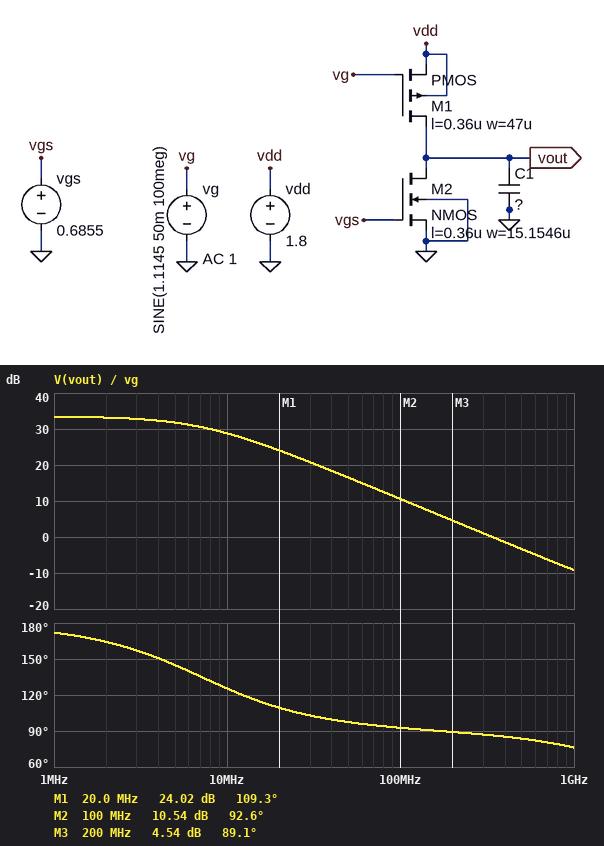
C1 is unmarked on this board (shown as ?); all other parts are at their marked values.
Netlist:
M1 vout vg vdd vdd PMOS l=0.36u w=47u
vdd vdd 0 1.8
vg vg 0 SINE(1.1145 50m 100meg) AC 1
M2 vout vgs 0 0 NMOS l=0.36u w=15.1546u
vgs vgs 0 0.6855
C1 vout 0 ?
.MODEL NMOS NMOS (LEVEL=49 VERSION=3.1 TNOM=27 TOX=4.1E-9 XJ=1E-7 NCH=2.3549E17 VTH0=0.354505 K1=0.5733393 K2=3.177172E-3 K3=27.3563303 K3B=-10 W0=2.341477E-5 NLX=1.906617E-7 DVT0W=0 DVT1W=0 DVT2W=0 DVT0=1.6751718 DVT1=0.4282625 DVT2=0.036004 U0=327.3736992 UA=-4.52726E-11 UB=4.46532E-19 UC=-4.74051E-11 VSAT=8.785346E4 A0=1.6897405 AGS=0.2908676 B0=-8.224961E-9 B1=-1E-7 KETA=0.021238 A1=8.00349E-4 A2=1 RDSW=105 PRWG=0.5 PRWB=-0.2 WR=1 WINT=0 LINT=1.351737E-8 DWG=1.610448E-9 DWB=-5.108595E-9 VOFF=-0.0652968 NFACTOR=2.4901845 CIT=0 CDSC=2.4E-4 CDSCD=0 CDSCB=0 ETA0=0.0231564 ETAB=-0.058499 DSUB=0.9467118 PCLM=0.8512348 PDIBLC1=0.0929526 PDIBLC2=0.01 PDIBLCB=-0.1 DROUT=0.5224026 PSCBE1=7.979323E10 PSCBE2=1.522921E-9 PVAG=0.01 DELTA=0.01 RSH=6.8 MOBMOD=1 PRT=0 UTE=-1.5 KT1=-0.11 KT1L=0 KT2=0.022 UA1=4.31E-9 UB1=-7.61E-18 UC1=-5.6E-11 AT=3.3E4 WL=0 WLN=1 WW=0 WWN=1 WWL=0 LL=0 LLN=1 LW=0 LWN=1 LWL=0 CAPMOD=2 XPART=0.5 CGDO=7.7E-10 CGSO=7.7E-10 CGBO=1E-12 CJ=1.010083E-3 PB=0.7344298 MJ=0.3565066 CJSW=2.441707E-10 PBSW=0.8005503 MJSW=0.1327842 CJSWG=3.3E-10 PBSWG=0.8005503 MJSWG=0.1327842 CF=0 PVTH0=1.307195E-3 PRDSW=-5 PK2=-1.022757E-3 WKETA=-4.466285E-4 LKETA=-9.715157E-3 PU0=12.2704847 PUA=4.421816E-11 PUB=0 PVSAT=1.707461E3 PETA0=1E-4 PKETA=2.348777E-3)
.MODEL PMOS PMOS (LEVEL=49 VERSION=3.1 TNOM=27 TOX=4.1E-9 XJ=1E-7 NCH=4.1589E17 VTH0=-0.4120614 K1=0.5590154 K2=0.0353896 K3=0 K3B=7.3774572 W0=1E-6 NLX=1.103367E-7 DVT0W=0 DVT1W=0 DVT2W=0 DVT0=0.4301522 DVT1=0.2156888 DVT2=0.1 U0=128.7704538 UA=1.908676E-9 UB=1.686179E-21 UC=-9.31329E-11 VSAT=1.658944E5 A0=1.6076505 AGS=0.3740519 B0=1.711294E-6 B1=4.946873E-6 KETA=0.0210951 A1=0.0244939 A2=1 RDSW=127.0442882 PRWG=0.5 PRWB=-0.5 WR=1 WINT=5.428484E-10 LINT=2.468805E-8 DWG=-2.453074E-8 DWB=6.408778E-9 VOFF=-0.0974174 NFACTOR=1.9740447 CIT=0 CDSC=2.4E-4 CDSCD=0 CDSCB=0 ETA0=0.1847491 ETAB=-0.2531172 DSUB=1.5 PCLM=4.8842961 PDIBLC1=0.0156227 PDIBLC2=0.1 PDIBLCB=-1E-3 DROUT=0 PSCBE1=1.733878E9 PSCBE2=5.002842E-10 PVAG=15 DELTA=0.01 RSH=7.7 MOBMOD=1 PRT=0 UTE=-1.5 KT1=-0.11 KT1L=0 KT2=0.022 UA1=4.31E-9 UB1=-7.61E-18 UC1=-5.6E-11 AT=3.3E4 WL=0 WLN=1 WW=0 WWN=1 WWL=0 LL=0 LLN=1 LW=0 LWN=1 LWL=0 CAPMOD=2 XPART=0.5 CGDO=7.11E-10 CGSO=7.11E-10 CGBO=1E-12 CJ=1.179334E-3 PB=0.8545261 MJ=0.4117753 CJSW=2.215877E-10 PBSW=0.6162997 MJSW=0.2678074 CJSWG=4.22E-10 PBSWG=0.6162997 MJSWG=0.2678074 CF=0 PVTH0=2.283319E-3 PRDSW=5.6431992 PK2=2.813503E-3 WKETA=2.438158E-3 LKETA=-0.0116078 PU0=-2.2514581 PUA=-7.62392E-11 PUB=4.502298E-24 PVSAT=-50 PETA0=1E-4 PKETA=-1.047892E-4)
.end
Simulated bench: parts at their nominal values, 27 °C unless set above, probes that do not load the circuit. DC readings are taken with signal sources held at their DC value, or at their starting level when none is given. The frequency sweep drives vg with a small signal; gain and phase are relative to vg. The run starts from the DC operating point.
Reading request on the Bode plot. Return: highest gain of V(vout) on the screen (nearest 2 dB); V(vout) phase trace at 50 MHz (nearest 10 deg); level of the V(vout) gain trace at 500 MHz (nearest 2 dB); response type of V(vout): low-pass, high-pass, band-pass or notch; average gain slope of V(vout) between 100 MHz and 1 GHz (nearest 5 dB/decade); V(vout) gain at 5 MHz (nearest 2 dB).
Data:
34 dB
100 deg
-4 dB
low-pass
-20 dB/decade
32 dB
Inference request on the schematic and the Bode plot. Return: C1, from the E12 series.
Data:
820 fF
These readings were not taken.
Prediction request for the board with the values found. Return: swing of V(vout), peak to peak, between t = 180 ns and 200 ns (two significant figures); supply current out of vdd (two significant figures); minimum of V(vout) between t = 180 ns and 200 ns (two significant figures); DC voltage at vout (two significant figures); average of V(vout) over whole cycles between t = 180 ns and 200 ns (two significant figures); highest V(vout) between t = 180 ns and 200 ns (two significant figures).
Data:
330 mV
220 µA
830 mV
880 mV
1.0 V
1.2 V
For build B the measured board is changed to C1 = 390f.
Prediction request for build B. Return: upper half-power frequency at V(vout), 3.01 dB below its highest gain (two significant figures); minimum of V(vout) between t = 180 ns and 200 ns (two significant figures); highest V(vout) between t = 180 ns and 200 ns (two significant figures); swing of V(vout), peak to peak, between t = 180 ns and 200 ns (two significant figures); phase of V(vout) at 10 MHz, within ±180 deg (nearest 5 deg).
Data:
14 MHz
680 mV
1.3 V
640 mV
145 deg
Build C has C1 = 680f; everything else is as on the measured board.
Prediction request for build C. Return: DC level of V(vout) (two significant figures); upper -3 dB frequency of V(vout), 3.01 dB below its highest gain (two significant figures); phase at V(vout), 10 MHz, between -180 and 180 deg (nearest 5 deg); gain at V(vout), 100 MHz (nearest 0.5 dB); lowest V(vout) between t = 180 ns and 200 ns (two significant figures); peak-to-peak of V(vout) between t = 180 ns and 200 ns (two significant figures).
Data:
880 mV
8.5 MHz
130 deg
12.0 dB
800 mV
390 mV
